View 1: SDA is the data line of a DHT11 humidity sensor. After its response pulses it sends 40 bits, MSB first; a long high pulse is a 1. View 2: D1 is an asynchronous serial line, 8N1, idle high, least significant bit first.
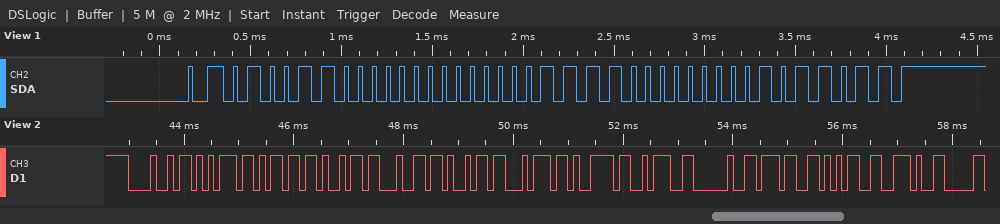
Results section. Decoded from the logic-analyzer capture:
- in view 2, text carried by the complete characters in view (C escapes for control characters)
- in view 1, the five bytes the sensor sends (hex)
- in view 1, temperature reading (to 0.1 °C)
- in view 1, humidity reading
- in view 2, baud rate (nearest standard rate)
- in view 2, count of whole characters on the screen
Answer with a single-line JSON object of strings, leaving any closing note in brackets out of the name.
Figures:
{"in view 2, text carried by the complete characters in view": "\"Humidity: 75.\"", "in view 1, the five bytes the sensor sends": "4C 00 0F 00 5B", "in view 1, temperature reading": "15.0 °C", "in view 1, humidity reading": "76 %", "in view 2, baud rate": "9600 baud", "in view 2, count of whole characters on the screen": "13"}
